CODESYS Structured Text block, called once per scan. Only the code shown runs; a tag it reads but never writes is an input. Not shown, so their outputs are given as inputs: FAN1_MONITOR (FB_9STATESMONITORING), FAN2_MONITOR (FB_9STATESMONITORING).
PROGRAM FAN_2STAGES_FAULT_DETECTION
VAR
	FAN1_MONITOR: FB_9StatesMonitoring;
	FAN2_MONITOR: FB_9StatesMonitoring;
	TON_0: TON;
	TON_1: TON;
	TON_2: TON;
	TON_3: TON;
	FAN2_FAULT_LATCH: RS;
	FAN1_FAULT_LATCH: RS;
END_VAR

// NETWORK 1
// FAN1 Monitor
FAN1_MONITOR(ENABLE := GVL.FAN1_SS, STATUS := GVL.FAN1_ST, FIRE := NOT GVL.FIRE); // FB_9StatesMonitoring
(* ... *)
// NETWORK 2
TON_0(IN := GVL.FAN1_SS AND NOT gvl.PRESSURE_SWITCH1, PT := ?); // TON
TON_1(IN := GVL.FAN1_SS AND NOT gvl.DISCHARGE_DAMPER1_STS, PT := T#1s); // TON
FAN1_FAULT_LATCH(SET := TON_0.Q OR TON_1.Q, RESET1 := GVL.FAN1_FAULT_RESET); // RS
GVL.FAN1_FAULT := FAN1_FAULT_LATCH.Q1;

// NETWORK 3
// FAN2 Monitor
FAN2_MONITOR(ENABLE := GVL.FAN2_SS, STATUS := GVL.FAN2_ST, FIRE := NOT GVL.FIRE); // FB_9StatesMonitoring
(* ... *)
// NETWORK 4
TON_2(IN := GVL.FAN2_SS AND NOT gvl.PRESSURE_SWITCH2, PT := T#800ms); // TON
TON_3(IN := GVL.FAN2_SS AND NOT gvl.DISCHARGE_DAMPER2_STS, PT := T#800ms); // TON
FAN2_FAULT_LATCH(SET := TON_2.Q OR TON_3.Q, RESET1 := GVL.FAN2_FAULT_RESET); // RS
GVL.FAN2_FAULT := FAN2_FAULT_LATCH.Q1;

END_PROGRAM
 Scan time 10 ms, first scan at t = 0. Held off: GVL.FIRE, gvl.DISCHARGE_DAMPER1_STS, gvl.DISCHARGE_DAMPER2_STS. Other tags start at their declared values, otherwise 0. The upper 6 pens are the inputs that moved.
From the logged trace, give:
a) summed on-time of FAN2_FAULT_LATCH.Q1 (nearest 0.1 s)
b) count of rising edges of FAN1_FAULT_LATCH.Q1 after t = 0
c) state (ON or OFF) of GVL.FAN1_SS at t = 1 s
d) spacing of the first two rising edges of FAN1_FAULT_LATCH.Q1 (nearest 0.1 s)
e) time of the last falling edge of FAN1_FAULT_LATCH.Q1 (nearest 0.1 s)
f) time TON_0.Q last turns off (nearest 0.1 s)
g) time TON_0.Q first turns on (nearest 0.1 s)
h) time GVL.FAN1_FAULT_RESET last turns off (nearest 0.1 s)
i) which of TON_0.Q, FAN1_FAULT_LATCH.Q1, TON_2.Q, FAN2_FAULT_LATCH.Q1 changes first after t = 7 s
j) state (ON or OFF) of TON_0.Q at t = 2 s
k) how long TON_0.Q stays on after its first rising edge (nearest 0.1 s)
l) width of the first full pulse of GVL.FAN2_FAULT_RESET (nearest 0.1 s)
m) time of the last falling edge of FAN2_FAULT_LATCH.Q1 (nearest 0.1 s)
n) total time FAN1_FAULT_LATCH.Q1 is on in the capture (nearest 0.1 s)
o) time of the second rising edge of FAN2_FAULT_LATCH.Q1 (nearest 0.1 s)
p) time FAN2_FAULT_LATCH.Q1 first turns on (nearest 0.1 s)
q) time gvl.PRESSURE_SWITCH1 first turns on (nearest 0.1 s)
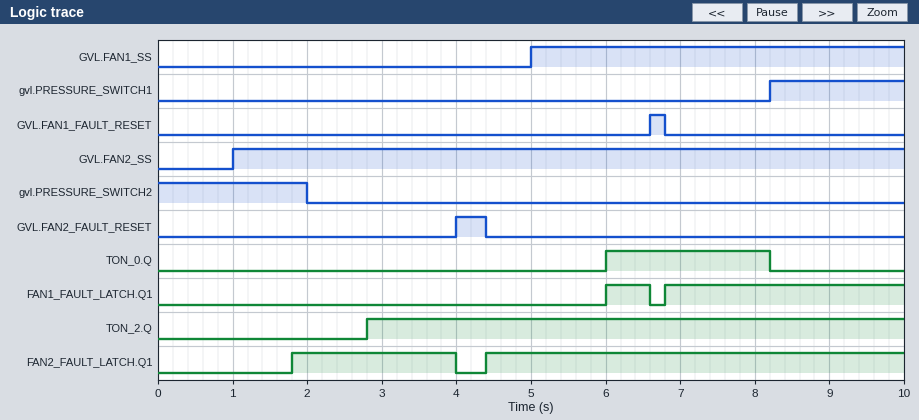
7.8 s
2
OFF
0.8 s
6.6 s
8.2 s
6.0 s
6.8 s
TON_0.Q
OFF
2.2 s
0.4 s
4.0 s
3.8 s
4.4 s
1.8 s
8.2 s
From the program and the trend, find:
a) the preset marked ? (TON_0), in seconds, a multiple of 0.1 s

1.0 s
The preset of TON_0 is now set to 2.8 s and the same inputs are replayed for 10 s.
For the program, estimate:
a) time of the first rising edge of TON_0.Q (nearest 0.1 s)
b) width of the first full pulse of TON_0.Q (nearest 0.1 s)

7.8 s
0.4 s
